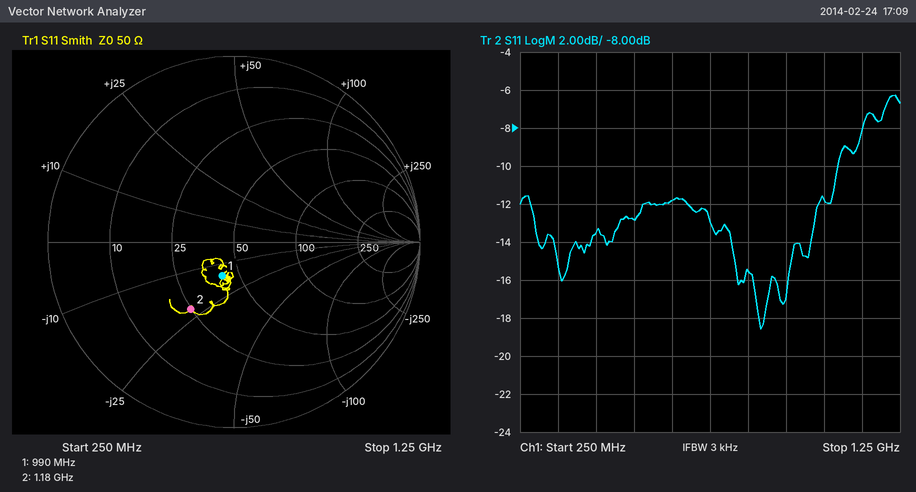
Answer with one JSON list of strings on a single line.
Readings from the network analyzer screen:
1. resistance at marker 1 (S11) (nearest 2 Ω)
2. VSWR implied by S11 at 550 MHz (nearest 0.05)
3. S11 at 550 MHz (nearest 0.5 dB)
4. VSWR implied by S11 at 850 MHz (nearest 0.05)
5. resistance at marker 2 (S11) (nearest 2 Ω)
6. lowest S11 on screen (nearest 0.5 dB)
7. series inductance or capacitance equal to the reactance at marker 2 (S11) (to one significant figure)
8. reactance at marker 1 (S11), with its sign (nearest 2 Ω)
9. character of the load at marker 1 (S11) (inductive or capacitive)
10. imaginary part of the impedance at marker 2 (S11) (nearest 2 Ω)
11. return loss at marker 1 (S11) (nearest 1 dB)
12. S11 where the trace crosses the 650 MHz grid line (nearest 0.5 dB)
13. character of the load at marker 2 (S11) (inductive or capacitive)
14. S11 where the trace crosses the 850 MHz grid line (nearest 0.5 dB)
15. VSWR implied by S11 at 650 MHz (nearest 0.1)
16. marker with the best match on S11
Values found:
["42 Ω", "1.60", "-13.0 dB", "1.40", "24 Ω", "-18.5 dB", "6 pF", "-16 Ω", "capacitive", "-22 Ω", "14 dB", "-12.0 dB", "capacitive", "-15.5 dB", "1.7", "marker 1"]
